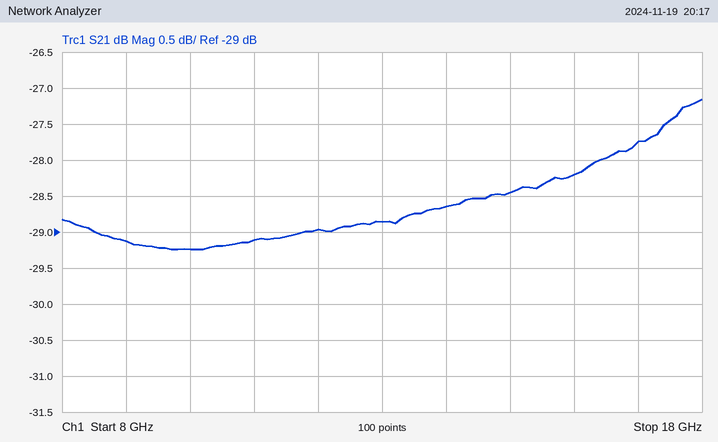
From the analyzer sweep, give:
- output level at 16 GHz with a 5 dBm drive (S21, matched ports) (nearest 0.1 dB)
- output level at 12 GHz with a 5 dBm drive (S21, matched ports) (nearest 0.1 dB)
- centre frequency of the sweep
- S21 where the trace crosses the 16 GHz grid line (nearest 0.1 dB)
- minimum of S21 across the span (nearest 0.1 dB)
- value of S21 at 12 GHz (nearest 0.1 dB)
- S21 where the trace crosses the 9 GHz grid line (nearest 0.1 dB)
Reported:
-23.2 dBm
-24.0 dBm
13 GHz
-28.2 dB
-29.2 dB
-29.0 dB
-29.1 dB
